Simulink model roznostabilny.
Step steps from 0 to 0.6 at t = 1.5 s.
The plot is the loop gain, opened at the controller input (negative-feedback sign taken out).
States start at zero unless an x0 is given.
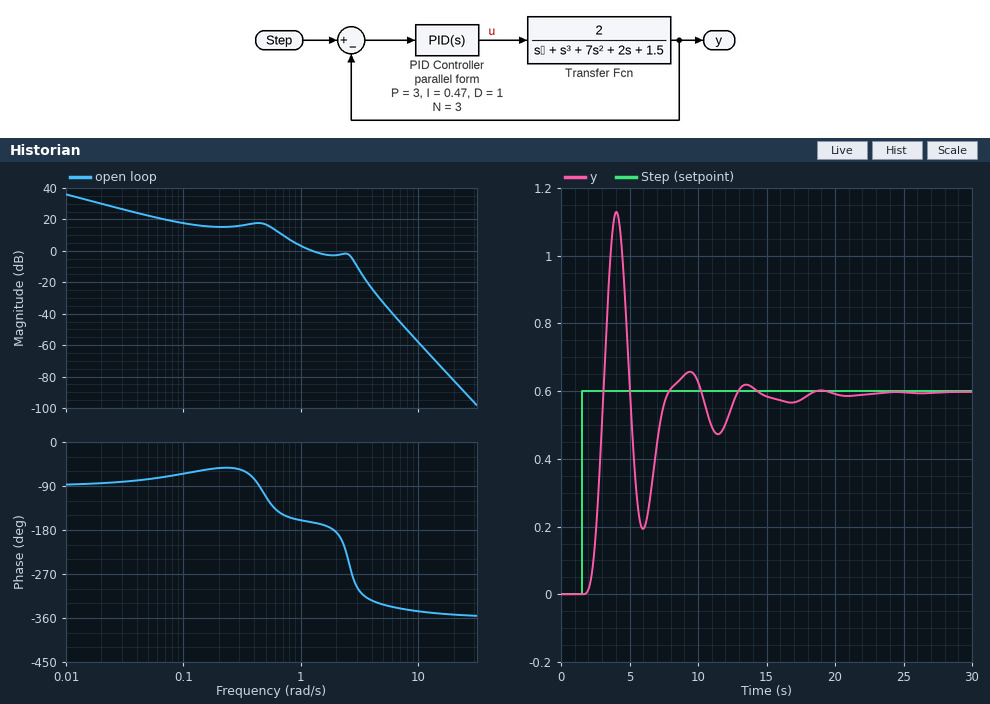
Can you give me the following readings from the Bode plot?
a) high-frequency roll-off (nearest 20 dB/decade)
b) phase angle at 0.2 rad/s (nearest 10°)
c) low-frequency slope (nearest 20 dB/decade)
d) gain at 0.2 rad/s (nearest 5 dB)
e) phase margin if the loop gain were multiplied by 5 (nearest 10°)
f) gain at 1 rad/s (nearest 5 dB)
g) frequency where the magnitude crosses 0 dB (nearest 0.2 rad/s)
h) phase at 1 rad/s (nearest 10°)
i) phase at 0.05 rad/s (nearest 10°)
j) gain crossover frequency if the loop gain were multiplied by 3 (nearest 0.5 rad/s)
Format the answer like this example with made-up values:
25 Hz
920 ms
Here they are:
-80 dB/decade
-50°
-20 dB/decade
15 dB
-130°
5 dB
1.2 rad/s
-160°
-80°
3.0 rad/s
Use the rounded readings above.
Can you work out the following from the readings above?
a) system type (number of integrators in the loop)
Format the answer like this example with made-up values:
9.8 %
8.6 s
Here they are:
1
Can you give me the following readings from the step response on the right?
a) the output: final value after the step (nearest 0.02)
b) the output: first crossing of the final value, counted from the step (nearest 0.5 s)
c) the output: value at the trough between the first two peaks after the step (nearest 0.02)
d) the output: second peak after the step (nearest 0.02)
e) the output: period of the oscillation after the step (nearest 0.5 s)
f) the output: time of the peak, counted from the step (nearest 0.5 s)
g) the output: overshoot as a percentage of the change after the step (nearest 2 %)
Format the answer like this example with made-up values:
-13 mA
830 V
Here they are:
0.60
1.5 s
0.20
0.66
5.5 s
2.5 s
88 %
